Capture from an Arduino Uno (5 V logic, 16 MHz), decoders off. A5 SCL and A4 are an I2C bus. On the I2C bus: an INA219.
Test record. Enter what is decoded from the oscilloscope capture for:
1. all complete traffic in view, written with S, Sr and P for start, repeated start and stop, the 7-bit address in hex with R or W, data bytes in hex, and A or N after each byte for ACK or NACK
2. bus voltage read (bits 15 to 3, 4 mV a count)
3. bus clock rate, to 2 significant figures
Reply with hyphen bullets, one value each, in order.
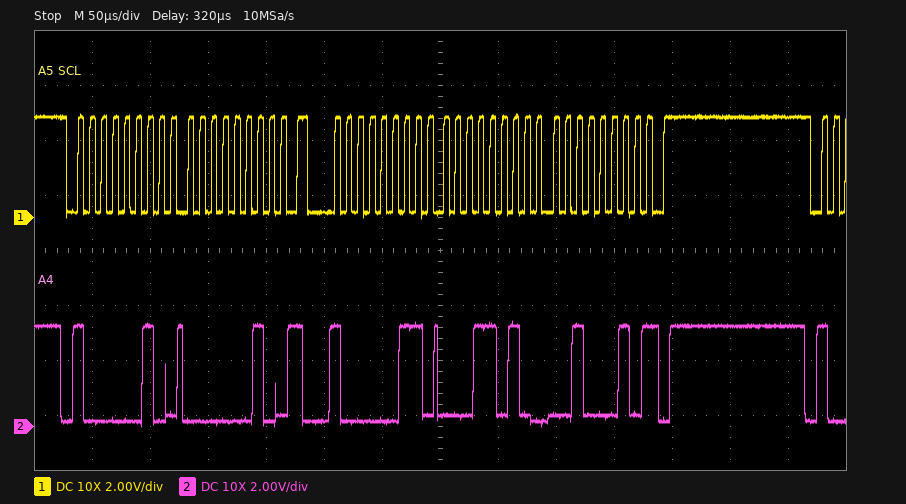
- S 41W A 02 A Sr 41R A 1A A 22 N P
- 3.344 V
- 100 kHz
